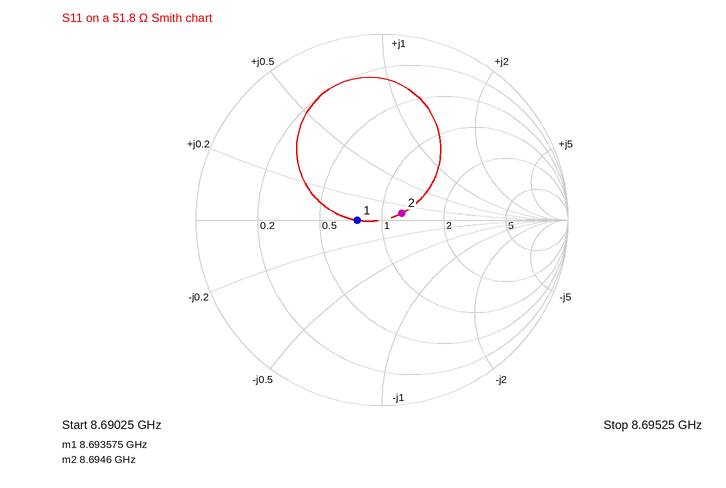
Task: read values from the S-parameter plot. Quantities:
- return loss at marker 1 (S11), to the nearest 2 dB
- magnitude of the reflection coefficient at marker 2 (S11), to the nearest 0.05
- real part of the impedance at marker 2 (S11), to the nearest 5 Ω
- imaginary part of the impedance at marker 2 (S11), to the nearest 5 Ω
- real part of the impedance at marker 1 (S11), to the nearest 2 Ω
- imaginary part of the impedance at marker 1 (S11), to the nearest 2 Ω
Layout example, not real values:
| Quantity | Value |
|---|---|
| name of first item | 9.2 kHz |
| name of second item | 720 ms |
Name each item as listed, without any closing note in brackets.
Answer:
| Quantity | Value |
|---|---|
| return loss at marker 1 (S11), to the nearest 2 dB | 18 dB |
| magnitude of the reflection coefficient at marker 2 (S11), to the nearest 0.05 | 0.10 |
| real part of the impedance at marker 2 (S11), to the nearest 5 Ω | 65 Ω |
| imaginary part of the impedance at marker 2 (S11), to the nearest 5 Ω | +5 Ω |
| real part of the impedance at marker 1 (S11), to the nearest 2 Ω | 40 Ω |
| imaginary part of the impedance at marker 1 (S11), to the nearest 2 Ω | 0 Ω |
